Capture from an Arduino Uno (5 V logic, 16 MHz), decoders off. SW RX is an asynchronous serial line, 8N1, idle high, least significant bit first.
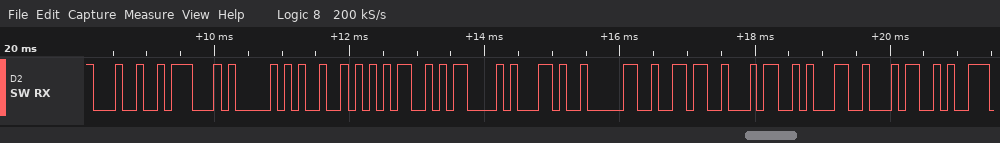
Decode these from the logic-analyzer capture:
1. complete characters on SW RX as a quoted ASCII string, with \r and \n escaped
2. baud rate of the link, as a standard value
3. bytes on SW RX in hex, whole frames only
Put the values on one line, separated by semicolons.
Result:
"$GPRMC,06414"; 9600 baud; 0x24 0x47 0x50 0x52 0x4D 0x43 0x2C 0x30 0x36 0x34 0x31 0x34
